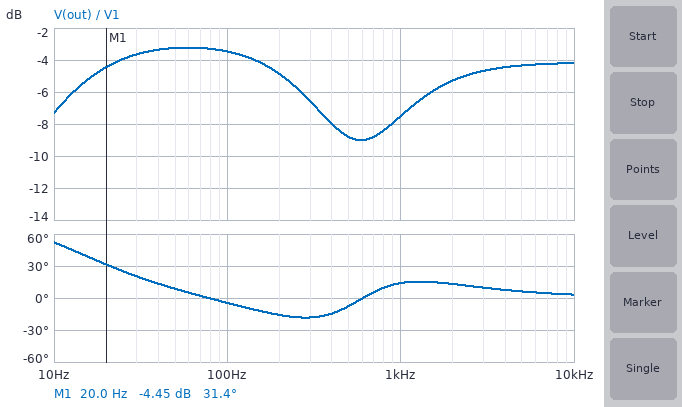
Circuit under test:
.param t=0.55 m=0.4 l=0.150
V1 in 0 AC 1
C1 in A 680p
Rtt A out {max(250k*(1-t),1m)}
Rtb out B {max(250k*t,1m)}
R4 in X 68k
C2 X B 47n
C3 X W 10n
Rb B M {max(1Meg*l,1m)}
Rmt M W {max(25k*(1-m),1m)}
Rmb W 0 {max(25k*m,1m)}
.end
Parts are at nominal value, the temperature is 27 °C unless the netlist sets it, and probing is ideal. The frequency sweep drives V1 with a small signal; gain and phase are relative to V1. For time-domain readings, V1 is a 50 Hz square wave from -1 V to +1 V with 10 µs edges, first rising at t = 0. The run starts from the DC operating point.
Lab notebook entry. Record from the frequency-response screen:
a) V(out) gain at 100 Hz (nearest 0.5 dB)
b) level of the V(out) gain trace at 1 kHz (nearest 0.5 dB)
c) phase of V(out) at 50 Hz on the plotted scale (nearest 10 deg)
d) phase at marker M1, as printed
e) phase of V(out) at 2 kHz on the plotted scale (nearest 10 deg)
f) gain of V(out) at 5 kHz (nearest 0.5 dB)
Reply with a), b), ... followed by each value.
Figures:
a) -3.5 dB
b) -7.5 dB
c) 10 deg
d) 31.4 deg
e) 10 deg
f) -4.5 dB
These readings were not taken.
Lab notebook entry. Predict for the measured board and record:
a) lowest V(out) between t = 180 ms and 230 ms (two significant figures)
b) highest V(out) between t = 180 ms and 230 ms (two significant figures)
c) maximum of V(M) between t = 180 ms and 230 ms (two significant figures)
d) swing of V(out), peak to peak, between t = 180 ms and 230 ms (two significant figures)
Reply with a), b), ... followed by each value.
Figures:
a) -850 mV
b) 850 mV
c) 250 mV
d) 1.7 V
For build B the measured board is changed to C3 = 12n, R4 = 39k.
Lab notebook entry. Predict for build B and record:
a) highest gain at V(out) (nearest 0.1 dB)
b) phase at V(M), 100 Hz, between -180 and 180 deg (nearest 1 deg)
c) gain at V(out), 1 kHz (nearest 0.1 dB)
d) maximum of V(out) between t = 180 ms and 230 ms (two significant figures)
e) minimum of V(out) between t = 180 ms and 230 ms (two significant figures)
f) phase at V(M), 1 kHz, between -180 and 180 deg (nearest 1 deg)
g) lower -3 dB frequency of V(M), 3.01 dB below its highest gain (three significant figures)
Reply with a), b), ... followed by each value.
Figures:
a) -2.0 dB
b) 18 deg
c) -6.7 dB
d) 1.0 V
e) -1.0 V
f) 12 deg
g) 289 Hz
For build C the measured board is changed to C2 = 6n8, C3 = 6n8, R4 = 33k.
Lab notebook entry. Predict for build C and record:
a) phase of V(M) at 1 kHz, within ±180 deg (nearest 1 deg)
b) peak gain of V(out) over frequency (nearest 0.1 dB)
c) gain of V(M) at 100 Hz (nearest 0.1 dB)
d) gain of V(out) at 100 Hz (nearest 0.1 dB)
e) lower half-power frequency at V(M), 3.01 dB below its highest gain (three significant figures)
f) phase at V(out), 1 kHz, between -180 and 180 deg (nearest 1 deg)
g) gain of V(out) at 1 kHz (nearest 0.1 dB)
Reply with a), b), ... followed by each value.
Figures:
a) 18 deg
b) -2.0 dB
c) -18.8 dB
d) -3.8 dB
e) 443 Hz
f) -3 deg
g) -4.4 dB
